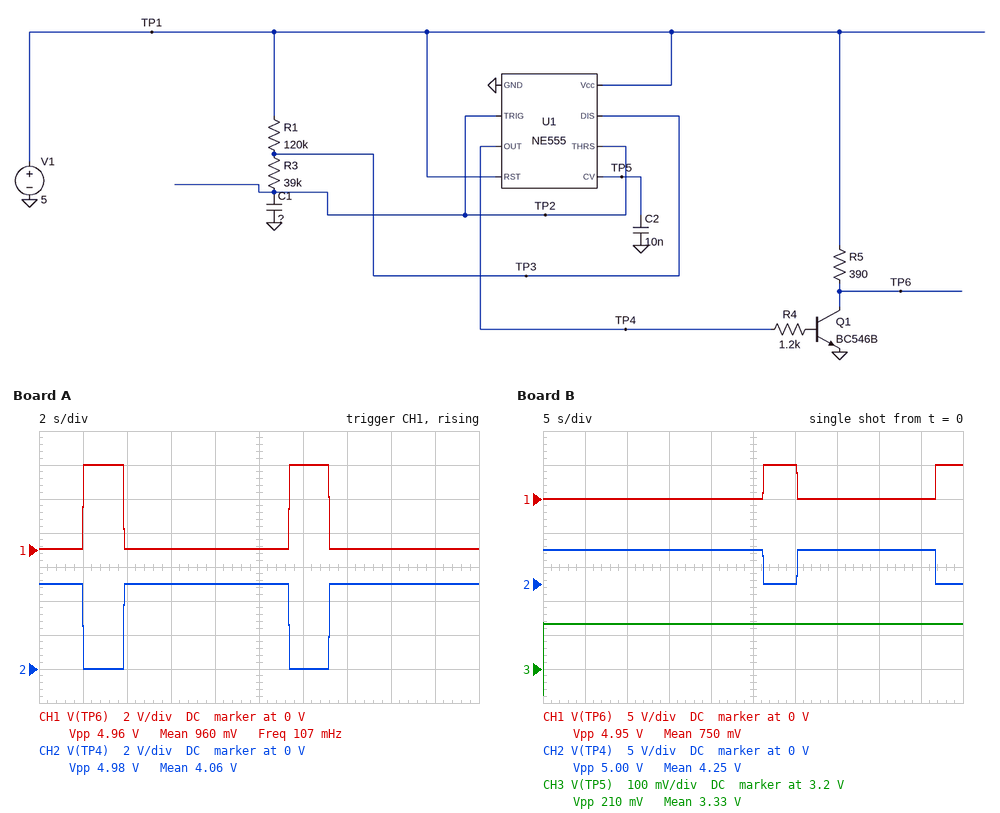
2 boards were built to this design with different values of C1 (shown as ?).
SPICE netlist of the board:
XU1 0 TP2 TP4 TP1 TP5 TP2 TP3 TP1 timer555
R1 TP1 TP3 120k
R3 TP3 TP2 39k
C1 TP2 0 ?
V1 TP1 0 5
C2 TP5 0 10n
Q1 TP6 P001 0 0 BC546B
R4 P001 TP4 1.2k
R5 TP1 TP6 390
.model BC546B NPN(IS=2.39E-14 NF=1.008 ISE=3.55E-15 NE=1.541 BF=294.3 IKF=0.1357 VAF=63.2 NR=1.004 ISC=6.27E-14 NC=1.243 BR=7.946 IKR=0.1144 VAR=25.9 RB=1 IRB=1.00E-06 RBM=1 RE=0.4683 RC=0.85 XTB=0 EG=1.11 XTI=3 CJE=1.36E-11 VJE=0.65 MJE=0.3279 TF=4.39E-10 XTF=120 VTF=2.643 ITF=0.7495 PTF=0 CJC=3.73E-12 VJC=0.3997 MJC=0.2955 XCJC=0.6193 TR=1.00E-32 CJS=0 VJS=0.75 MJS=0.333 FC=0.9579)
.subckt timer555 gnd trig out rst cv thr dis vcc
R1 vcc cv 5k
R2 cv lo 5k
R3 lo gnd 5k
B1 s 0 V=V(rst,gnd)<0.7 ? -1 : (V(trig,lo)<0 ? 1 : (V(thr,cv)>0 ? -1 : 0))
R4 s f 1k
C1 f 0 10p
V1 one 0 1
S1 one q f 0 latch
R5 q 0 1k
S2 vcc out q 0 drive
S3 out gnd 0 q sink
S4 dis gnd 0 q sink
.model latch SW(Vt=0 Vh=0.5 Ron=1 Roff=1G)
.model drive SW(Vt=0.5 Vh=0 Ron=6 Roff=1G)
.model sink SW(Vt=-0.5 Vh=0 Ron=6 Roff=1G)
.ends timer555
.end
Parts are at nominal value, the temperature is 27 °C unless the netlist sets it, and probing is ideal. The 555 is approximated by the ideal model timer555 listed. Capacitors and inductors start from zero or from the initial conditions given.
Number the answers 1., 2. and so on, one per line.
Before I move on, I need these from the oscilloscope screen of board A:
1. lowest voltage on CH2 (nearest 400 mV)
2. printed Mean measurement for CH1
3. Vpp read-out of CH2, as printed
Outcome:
1. 0 V
2. 960 mV
3. 4.98 V
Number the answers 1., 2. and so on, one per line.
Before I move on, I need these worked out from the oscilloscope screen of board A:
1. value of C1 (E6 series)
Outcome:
1. 68 µF
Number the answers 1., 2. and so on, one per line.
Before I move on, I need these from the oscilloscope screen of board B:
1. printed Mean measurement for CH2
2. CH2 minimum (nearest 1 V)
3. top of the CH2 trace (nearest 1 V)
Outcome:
1. 4.25 V
2. 0 V
3. 5 V
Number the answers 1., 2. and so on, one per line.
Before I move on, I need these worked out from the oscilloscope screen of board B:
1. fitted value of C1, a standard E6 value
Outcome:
1. 150 µF
